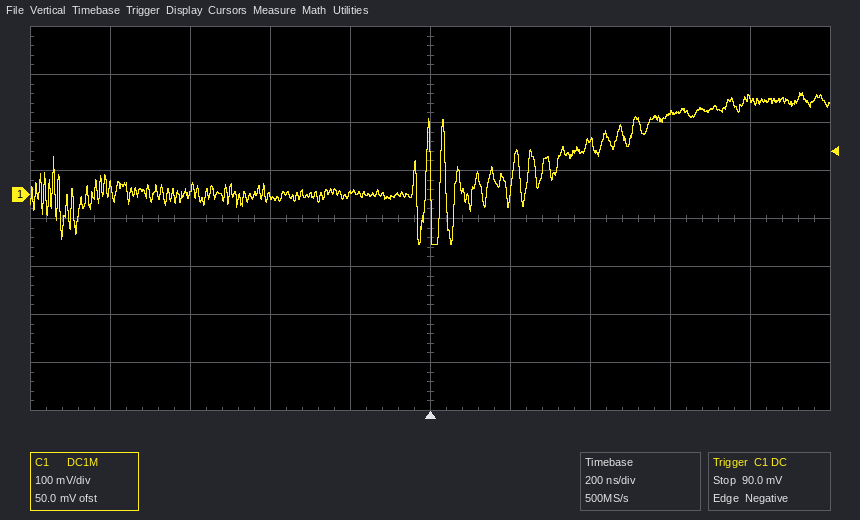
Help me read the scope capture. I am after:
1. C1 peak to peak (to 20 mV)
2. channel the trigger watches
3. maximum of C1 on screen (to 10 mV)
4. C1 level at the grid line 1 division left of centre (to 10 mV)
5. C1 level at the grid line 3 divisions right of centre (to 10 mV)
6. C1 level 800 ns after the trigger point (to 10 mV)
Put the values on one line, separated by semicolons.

320 mV; C1; 210 mV; 0 mV; 170 mV; 200 mV
